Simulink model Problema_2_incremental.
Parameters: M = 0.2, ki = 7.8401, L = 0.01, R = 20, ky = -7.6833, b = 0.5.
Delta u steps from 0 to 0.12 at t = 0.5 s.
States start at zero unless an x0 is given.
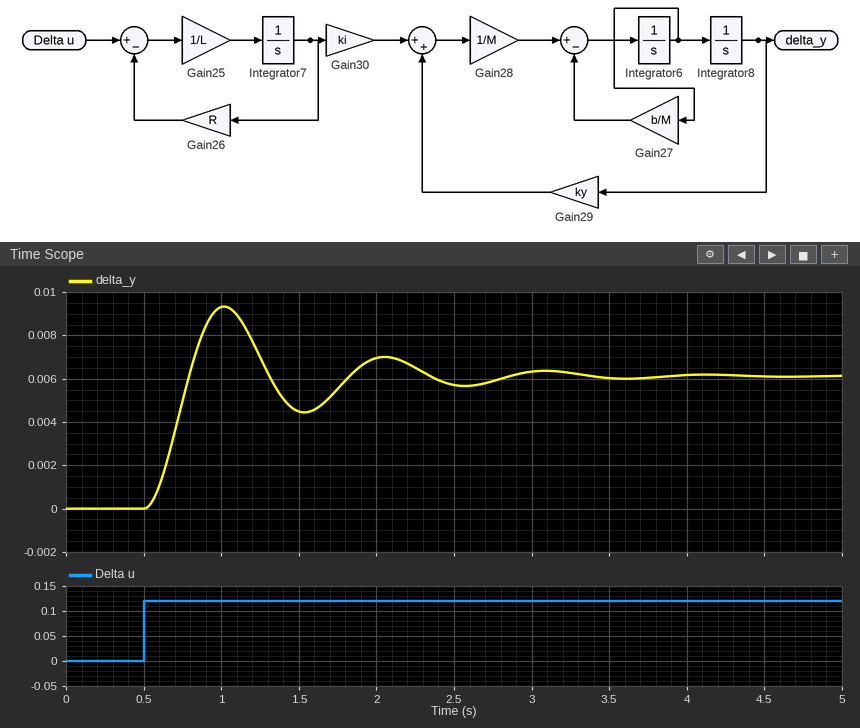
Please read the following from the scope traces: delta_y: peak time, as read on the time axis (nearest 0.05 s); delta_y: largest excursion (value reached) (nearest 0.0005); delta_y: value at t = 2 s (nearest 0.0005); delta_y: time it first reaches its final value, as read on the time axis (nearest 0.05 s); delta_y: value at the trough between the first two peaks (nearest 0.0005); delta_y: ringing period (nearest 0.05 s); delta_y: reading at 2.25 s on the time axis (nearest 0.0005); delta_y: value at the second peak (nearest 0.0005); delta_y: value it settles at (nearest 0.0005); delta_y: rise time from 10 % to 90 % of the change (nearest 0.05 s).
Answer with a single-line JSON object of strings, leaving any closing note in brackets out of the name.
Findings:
{"delta_y: peak time, as read on the time axis": "1.00 s", "delta_y: largest excursion (value reached)": "0.0095", "delta_y: value at t = 2 s": "0.0070", "delta_y: time it first reaches its final value, as read on the time axis": "0.80 s", "delta_y: value at the trough between the first two peaks": "0.0045", "delta_y: ringing period": "1.05 s", "delta_y: reading at 2.25 s on the time axis": "0.0065", "delta_y: value at the second peak": "0.0070", "delta_y: value it settles at": "0.0060", "delta_y: rise time from 10 % to 90 % of the change": "0.20 s"}
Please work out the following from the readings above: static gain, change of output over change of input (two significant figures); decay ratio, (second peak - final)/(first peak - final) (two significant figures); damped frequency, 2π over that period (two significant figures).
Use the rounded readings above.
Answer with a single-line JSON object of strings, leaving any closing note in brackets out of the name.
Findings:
{"static gain, change of output over change of input": "0.050", "decay ratio, (second peak - final)/(first peak - final)": "0.29", "damped frequency, 2π over that period": "6.0 rad/s"}
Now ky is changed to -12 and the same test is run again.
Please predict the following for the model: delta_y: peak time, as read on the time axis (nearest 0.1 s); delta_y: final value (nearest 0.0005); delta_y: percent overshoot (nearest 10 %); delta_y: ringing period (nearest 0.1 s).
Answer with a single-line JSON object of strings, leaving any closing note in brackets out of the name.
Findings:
{"delta_y: peak time, as read on the time axis": "0.9 s", "delta_y: final value": "0.0040", "delta_y: percent overshoot": "60 %", "delta_y: ringing period": "0.8 s"}
